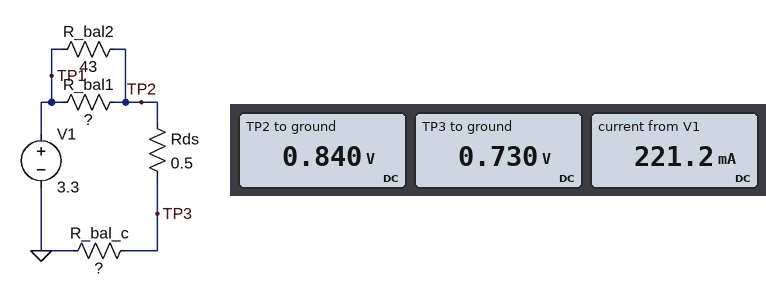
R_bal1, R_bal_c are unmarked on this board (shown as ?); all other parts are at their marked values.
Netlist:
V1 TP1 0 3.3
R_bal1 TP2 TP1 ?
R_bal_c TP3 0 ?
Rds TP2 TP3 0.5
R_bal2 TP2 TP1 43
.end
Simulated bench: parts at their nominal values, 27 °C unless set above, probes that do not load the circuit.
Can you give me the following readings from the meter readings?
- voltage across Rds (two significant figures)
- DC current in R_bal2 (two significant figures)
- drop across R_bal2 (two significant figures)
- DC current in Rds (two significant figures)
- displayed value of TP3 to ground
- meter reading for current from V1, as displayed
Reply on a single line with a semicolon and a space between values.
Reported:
110 mV; 57 mA; 2.5 V; 220 mA; 0.730 V; 221.2 mA
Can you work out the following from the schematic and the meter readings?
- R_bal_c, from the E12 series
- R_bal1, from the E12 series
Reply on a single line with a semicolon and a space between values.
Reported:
3.3 Ω; 15 Ω
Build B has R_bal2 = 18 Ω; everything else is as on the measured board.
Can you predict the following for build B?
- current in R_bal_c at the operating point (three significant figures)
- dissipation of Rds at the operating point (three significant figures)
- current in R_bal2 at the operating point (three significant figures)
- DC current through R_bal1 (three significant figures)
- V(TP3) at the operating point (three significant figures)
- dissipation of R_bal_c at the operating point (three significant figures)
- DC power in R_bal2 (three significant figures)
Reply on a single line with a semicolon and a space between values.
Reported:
275 mA; 37.9 mW; 125 mA; 150 mA; 909 mV; 250 mW; 282 mW
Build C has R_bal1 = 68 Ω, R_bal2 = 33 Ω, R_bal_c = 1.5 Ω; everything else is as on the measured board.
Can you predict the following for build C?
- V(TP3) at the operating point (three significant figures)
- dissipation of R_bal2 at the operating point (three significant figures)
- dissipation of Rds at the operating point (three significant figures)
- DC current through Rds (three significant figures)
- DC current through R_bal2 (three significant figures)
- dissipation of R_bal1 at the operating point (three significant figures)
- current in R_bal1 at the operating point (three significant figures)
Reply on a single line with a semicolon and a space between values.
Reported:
204 mV; 278 mW; 9.28 mW; 136 mA; 91.7 mA; 135 mW; 44.5 mA
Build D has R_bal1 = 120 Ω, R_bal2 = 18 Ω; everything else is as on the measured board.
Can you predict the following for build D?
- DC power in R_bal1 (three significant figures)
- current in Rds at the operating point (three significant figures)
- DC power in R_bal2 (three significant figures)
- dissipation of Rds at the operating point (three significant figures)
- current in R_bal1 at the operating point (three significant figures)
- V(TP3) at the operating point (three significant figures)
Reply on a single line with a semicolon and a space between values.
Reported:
58.8 mW; 170 mA; 392 mW; 14.4 mW; 22.1 mA; 560 mV
